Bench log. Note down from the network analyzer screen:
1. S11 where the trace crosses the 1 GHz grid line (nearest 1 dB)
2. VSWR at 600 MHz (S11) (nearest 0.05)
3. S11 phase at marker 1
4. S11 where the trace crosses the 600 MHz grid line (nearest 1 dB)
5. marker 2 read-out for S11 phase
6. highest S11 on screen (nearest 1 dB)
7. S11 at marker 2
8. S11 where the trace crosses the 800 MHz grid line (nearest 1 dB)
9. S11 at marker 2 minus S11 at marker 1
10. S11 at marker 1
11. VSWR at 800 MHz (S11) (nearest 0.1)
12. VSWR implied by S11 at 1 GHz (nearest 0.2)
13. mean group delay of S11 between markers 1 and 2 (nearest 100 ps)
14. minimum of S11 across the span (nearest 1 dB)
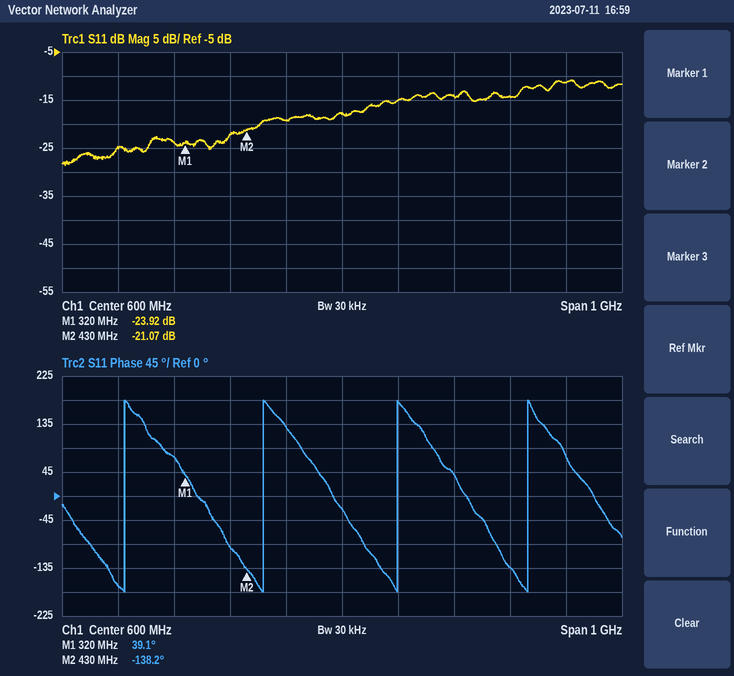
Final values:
-11 dB
1.30
39.1°
-18 dB
-138.2°
-11 dB
-21.07 dB
-14 dB
2.85 dB
-23.92 dB
1.5
1.8
4.5 ns
-29 dB
